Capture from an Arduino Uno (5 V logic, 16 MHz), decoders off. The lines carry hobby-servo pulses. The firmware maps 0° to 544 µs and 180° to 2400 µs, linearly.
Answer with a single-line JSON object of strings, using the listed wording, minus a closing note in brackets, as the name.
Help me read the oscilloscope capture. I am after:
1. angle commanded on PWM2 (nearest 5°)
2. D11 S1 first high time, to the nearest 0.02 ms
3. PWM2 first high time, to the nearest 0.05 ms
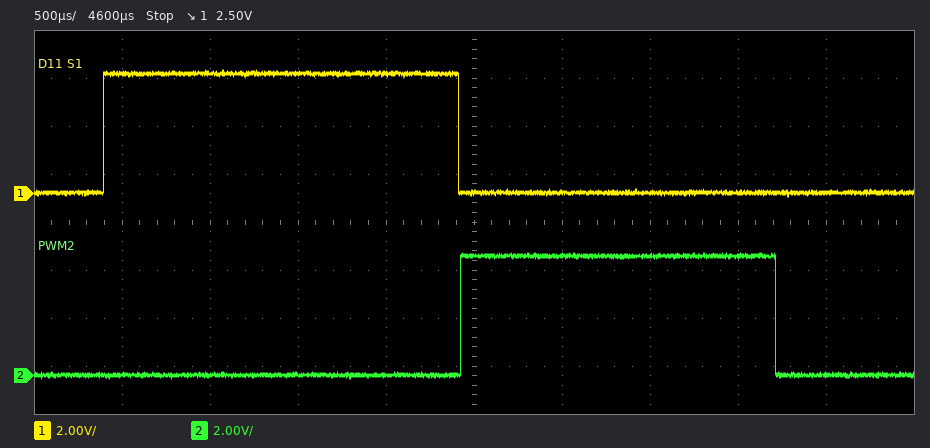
{"angle commanded on PWM2": "120°", "D11 S1 first high time, to the nearest 0.02 ms": "2.02 ms", "PWM2 first high time, to the nearest 0.05 ms": "1.80 ms"}
